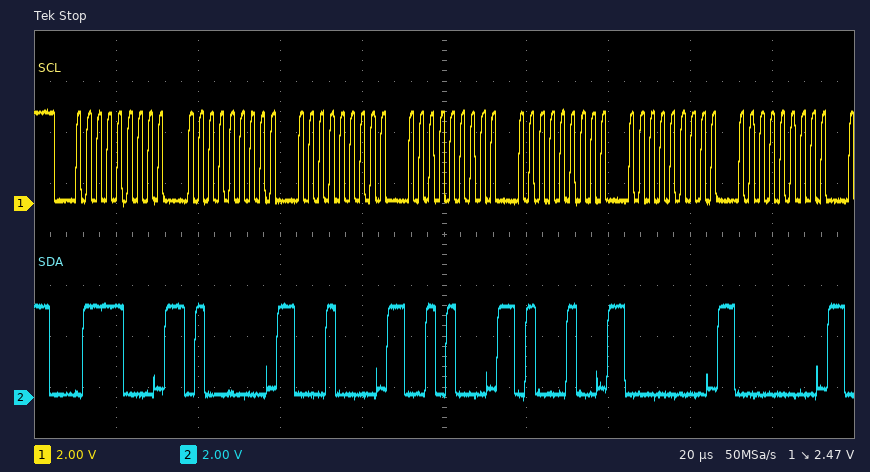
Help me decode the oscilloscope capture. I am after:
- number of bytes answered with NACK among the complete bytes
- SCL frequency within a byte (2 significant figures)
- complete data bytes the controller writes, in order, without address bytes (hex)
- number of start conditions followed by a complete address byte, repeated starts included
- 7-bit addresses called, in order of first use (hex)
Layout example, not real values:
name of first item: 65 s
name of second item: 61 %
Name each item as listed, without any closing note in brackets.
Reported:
number of bytes answered with NACK among the complete bytes: 0
SCL frequency within a byte: 400 kHz
complete data bytes the controller writes, in order, without address bytes: 40 10 28 44 00 00
number of start conditions followed by a complete address byte, repeated starts included: 1
7-bit addresses called, in order of first use: 0x3C
